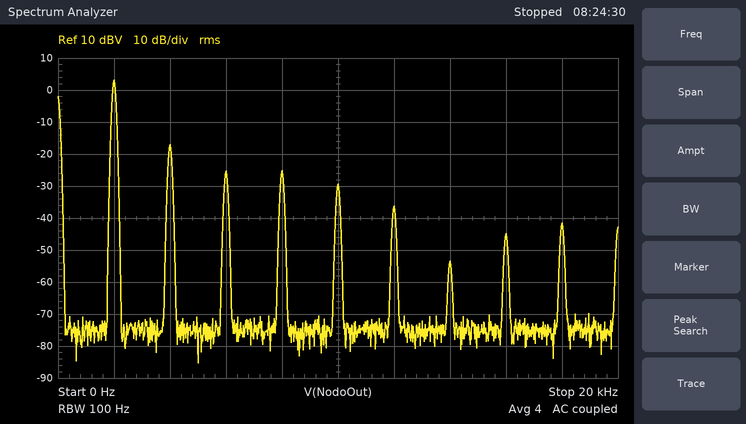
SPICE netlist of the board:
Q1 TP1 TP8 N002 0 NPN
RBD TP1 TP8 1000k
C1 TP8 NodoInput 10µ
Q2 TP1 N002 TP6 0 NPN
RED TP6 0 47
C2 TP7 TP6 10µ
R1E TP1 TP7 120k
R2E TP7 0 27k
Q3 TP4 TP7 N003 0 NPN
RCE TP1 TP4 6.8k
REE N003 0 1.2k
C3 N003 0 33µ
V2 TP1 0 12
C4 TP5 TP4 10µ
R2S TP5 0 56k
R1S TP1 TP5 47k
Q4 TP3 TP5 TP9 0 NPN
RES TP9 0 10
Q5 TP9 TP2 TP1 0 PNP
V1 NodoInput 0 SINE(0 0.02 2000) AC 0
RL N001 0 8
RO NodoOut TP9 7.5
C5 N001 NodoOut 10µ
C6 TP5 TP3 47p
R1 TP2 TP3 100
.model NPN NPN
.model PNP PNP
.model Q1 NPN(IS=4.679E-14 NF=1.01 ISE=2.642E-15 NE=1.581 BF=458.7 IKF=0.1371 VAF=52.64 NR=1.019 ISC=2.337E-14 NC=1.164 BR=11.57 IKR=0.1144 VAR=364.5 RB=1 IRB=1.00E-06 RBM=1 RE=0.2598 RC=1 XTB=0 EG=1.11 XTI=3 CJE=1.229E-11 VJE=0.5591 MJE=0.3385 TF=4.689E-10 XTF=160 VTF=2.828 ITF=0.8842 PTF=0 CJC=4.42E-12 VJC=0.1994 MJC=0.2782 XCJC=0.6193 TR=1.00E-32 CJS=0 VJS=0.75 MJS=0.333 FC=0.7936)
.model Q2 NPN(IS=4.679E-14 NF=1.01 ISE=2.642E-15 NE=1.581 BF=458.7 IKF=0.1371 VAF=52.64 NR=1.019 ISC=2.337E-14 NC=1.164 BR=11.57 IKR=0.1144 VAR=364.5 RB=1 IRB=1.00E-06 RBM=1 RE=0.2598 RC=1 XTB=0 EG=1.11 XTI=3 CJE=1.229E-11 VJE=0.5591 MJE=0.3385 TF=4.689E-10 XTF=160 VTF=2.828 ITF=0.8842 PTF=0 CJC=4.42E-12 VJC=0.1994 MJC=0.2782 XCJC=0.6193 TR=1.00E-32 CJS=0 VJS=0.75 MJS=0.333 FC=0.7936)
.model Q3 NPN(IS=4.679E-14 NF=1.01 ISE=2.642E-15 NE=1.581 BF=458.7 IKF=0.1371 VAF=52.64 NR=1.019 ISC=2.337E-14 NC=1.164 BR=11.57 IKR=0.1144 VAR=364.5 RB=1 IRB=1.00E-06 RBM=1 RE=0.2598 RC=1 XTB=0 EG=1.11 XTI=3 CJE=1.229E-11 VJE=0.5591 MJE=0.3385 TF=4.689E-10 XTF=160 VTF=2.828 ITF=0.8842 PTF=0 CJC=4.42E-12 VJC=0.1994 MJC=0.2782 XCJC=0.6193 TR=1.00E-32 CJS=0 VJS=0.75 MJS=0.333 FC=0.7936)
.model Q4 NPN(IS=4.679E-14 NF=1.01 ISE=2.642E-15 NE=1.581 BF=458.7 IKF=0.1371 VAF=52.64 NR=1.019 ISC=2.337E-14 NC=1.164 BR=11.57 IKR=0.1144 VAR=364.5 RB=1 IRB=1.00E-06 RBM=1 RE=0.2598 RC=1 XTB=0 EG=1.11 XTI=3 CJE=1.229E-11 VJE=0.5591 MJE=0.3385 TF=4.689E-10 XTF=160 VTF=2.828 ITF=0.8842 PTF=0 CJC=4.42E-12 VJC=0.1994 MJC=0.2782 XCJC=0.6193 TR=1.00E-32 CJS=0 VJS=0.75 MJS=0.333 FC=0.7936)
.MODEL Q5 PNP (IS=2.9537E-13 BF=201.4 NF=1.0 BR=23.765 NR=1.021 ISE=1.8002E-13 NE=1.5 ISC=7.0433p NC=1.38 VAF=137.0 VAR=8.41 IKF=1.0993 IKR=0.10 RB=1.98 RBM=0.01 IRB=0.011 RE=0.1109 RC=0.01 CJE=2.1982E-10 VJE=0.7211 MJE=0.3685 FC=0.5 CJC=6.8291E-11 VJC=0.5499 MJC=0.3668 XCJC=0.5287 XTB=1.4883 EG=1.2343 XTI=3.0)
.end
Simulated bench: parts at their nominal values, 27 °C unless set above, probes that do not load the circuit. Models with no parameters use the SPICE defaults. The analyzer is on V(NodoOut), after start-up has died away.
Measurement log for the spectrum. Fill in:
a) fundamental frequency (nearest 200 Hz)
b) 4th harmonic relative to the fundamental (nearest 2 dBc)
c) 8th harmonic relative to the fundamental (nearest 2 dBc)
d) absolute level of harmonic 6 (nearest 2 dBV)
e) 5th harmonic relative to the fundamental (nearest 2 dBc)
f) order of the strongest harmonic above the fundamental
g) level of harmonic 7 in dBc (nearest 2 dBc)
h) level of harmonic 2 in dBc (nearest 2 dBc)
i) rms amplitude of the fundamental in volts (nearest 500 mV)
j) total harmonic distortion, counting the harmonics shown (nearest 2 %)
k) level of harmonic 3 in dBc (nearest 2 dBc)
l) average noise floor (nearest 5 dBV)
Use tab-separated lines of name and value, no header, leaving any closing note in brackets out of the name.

fundamental frequency	2.0 kHz
4th harmonic relative to the fundamental	-28 dBc
8th harmonic relative to the fundamental	-48 dBc
absolute level of harmonic 6	-36 dBV
5th harmonic relative to the fundamental	-32 dBc
order of the strongest harmonic above the fundamental	2
level of harmonic 7 in dBc	-56 dBc
level of harmonic 2 in dBc	-20 dBc
rms amplitude of the fundamental in volts	1.5 V
total harmonic distortion, counting the harmonics shown	12 %
level of harmonic 3 in dBc	-28 dBc
average noise floor	-75 dBV
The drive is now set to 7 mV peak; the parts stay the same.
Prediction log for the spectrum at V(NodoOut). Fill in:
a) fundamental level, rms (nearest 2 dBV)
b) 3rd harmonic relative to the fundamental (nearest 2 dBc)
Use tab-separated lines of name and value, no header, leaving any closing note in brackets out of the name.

fundamental level, rms	-4 dBV
3rd harmonic relative to the fundamental	-54 dBc
